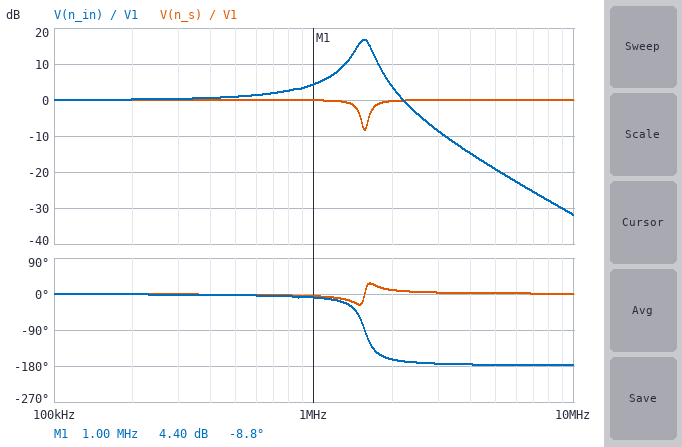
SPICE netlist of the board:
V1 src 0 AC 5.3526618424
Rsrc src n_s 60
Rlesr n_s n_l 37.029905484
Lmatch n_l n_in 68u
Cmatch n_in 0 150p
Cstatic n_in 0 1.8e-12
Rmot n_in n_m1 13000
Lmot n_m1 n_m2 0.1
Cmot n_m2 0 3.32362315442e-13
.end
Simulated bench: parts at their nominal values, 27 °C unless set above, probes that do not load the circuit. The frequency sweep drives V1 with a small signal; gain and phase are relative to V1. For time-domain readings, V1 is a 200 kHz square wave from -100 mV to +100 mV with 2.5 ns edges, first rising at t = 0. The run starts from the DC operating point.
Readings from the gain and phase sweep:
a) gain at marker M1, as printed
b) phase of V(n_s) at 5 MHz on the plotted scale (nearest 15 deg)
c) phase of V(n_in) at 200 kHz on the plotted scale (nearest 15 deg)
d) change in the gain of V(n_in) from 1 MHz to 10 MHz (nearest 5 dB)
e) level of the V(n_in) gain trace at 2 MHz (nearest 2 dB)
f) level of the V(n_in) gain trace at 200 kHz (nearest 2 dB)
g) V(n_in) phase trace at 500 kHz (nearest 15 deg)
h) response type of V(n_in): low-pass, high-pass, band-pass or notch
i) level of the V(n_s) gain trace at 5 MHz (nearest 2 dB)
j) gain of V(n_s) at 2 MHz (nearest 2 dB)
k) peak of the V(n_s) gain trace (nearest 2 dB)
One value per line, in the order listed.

4.40 dB
0 deg
0 deg
-35 dB
4 dB
0 dB
0 deg
low-pass
0 dB
0 dB
0 dB
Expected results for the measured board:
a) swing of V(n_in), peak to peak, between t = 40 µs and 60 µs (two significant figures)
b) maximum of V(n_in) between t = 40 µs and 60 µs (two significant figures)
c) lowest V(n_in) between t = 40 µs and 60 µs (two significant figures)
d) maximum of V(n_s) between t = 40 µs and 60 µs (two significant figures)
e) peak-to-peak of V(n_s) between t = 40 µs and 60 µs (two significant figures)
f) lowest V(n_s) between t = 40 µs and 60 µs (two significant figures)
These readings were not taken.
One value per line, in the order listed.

480 mV
240 mV
-240 mV
110 mV
220 mV
-110 mV
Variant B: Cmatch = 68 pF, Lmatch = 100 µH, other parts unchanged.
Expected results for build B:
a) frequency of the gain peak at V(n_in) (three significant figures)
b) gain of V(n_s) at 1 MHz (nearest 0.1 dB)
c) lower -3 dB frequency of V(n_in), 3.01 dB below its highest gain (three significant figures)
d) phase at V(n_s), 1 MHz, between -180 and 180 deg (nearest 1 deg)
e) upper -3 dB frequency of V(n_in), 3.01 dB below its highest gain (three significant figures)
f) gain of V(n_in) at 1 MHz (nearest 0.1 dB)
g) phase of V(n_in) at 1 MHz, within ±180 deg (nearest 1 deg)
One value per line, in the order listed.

1.90 MHz
0 dB
1.82 MHz
-2 deg
1.98 MHz
2.7 dB
-3 deg
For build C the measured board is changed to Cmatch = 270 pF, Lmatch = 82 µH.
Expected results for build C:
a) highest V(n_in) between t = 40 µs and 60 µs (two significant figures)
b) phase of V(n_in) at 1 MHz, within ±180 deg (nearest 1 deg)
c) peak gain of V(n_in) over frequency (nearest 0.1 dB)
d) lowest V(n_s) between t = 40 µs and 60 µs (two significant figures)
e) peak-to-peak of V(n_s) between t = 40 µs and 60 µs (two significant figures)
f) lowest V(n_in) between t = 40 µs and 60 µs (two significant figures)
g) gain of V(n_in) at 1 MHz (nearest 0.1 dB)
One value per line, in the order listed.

270 mV
-53 deg
15.1 dB
-120 mV
230 mV
-270 mV
13.7 dB
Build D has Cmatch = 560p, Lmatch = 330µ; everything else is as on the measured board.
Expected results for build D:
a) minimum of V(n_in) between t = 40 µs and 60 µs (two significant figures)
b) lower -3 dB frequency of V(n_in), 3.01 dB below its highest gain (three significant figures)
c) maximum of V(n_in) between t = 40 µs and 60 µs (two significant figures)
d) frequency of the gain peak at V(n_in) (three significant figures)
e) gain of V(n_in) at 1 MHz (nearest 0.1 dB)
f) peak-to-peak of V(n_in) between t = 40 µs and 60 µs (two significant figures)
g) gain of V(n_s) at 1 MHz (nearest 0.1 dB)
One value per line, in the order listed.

-200 mV
344 kHz
200 mV
368 kHz
-16.0 dB
400 mV
0 dB
